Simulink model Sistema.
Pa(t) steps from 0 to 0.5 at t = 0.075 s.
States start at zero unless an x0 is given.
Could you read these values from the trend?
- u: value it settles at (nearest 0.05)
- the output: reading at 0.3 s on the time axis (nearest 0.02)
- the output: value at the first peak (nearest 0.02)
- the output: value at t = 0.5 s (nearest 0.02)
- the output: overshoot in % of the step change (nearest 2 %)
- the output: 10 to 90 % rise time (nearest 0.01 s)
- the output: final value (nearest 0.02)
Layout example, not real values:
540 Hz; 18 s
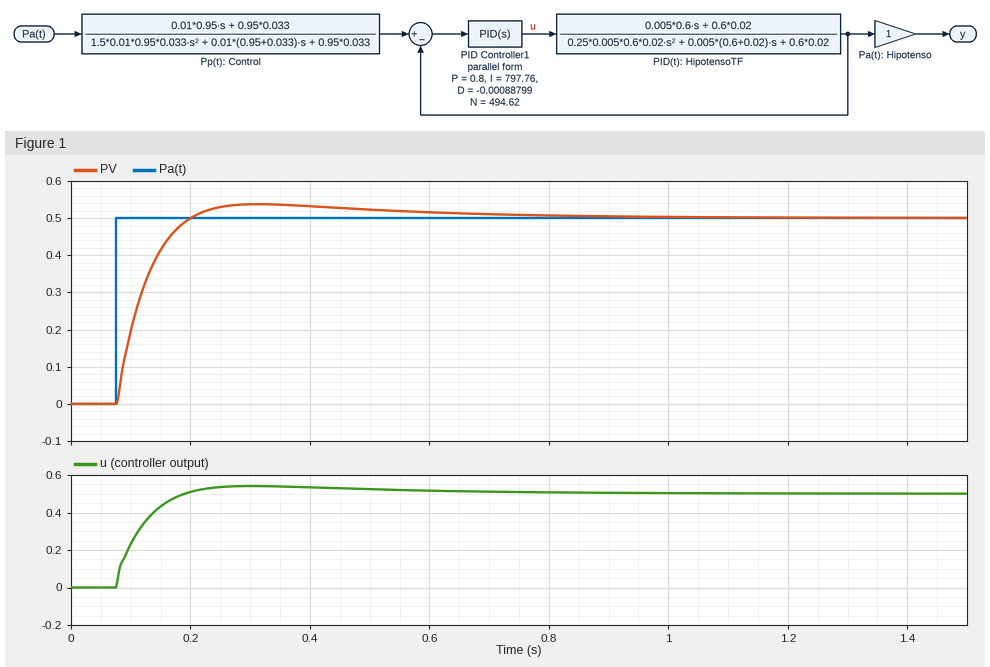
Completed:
0.50; 0.54; 0.54; 0.52; 8 %; 0.08 s; 0.50
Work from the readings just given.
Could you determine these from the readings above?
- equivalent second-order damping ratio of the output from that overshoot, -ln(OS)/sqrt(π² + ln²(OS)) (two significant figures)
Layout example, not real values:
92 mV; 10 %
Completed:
0.63
